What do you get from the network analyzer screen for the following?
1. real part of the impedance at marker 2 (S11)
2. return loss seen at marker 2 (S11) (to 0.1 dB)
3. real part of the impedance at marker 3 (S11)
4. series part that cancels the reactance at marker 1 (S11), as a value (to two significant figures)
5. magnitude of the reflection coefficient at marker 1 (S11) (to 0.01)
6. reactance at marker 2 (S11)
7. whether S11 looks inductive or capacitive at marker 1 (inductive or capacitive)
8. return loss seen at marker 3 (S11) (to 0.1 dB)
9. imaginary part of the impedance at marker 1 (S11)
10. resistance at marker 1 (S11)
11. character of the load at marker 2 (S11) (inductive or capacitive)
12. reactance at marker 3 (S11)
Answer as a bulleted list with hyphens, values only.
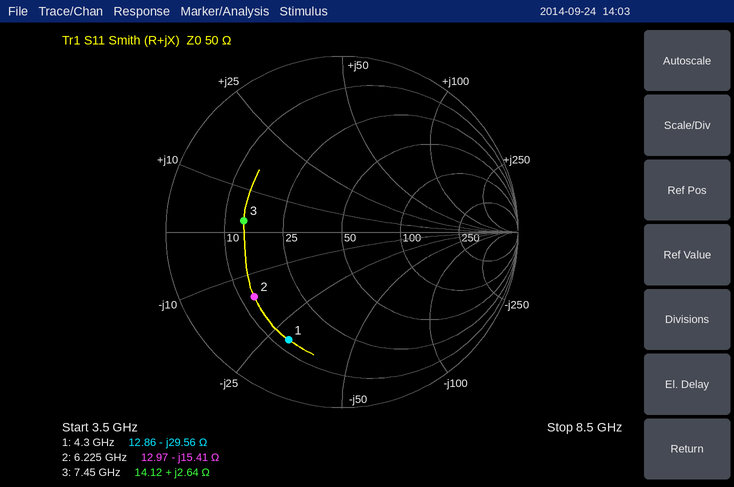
- 12.97 Ω
- 4.2 dB
- 14.12 Ω
- 1.1 nH
- 0.68
- -15.41 Ω
- capacitive
- 5.0 dB
- -29.56 Ω
- 12.86 Ω
- capacitive
- +2.64 Ω
